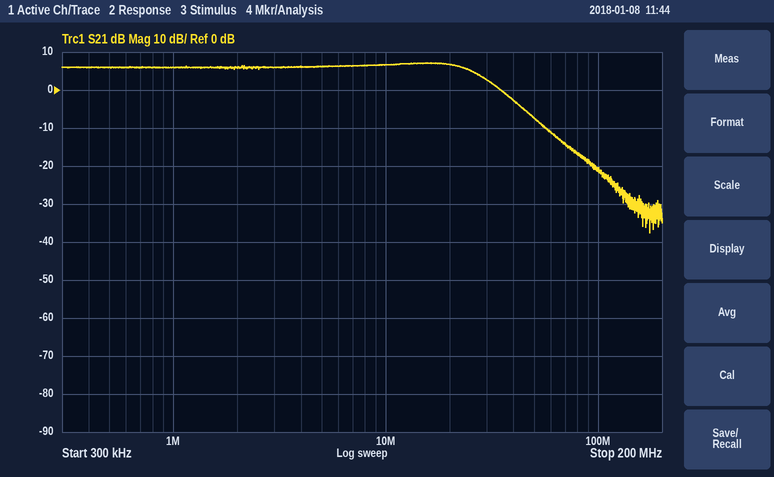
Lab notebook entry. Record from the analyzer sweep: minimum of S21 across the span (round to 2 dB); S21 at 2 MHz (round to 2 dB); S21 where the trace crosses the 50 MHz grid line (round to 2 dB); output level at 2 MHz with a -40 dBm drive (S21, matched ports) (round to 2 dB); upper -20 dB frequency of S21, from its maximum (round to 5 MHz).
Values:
-38 dB
6 dB
-8 dB
-34 dBm
65 MHz
